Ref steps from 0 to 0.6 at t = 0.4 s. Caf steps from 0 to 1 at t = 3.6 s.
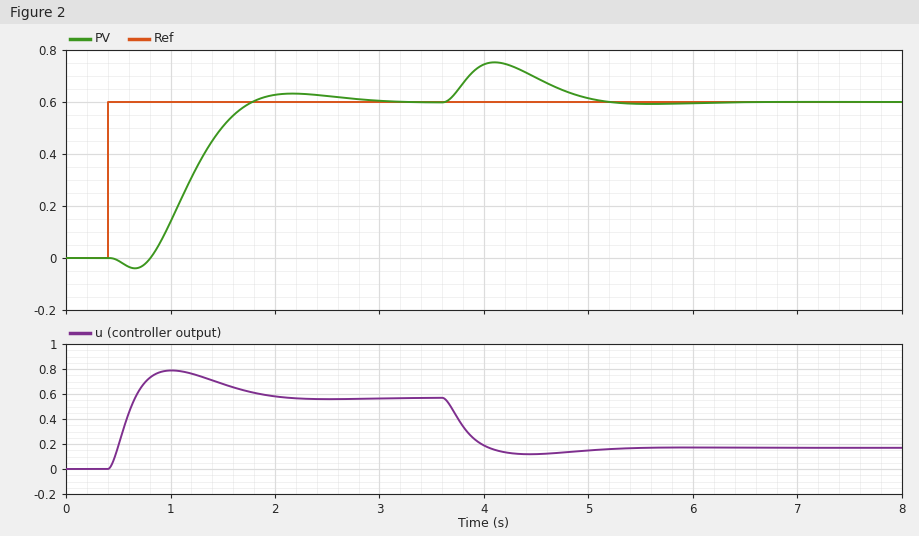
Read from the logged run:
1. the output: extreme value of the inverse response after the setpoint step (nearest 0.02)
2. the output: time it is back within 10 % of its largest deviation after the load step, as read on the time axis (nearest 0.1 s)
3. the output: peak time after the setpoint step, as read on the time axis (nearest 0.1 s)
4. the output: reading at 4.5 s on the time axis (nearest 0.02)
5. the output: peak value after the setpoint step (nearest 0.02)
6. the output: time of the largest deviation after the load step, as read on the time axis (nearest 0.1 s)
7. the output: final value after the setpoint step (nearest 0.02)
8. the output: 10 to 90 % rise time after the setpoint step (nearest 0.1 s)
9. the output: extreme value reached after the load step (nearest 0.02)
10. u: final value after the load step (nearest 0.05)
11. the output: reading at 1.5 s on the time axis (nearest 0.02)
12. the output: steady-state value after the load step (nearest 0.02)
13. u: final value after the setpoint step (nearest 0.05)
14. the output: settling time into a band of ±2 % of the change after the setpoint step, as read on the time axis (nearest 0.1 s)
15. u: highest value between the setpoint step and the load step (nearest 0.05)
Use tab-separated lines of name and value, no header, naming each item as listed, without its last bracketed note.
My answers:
the output: extreme value of the inverse response after the setpoint step	-0.04
the output: time it is back within 10 % of its largest deviation after the load step, as read on the time axis	5.0 s
the output: peak time after the setpoint step, as read on the time axis	2.2 s
the output: reading at 4.5 s on the time axis	0.70
the output: peak value after the setpoint step	0.64
the output: time of the largest deviation after the load step, as read on the time axis	4.1 s
the output: final value after the setpoint step	0.60
the output: 10 to 90 % rise time after the setpoint step	0.7 s
the output: extreme value reached after the load step	0.76
u: final value after the load step	0.15
the output: reading at 1.5 s on the time axis	0.50
the output: steady-state value after the load step	0.60
u: final value after the setpoint step	0.55
the output: settling time into a band of ±2 % of the change after the setpoint step, as read on the time axis	2.8 s
u: highest value between the setpoint step and the load step	0.80
